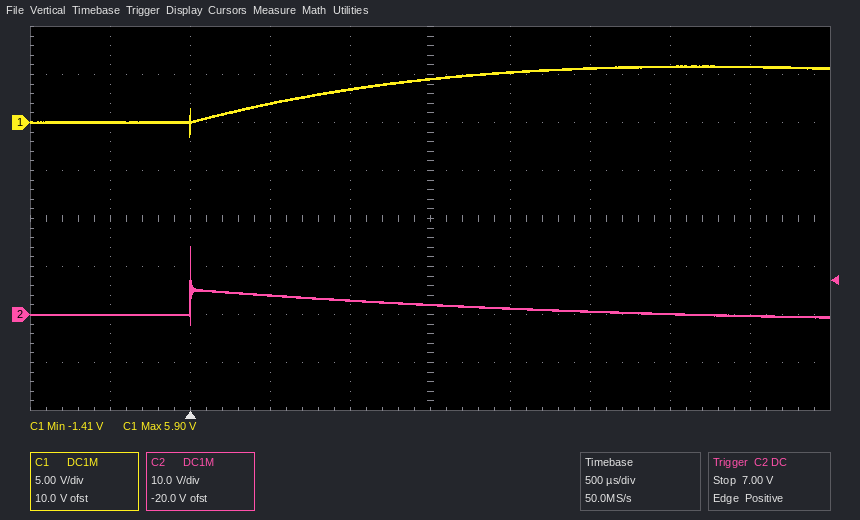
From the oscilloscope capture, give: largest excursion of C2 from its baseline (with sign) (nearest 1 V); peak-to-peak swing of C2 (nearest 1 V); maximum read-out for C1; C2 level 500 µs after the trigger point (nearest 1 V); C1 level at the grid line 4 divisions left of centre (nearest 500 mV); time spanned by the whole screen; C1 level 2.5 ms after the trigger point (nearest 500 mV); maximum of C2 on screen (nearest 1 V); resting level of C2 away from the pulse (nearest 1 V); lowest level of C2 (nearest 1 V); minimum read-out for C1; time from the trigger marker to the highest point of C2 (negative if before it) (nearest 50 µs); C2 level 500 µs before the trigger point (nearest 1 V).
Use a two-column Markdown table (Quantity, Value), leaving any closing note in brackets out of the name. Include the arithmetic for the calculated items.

| Quantity | Value |
|---|---|
| largest excursion of C2 from its baseline (with sign) | 14 V − (0 V) = +14 V |
| peak-to-peak swing of C2 | 14 V − (-2 V) = 16 V |
| maximum read-out for C1 | 5.90 V |
| C2 level 500 µs after the trigger point | 4 V |
| C1 level at the grid line 4 divisions left of centre | 0.0 V |
| time spanned by the whole screen | 5 ms |
| C1 level 2.5 ms after the trigger point | 5.5 V |
| maximum of C2 on screen | 14 V |
| resting level of C2 away from the pulse | 0 V |
| lowest level of C2 | -2 V |
| minimum read-out for C1 | -1.41 V |
| time from the trigger marker to the highest point of C2 (negative if before it) | 0 µs |
| C2 level 500 µs before the trigger point | 0 V |
